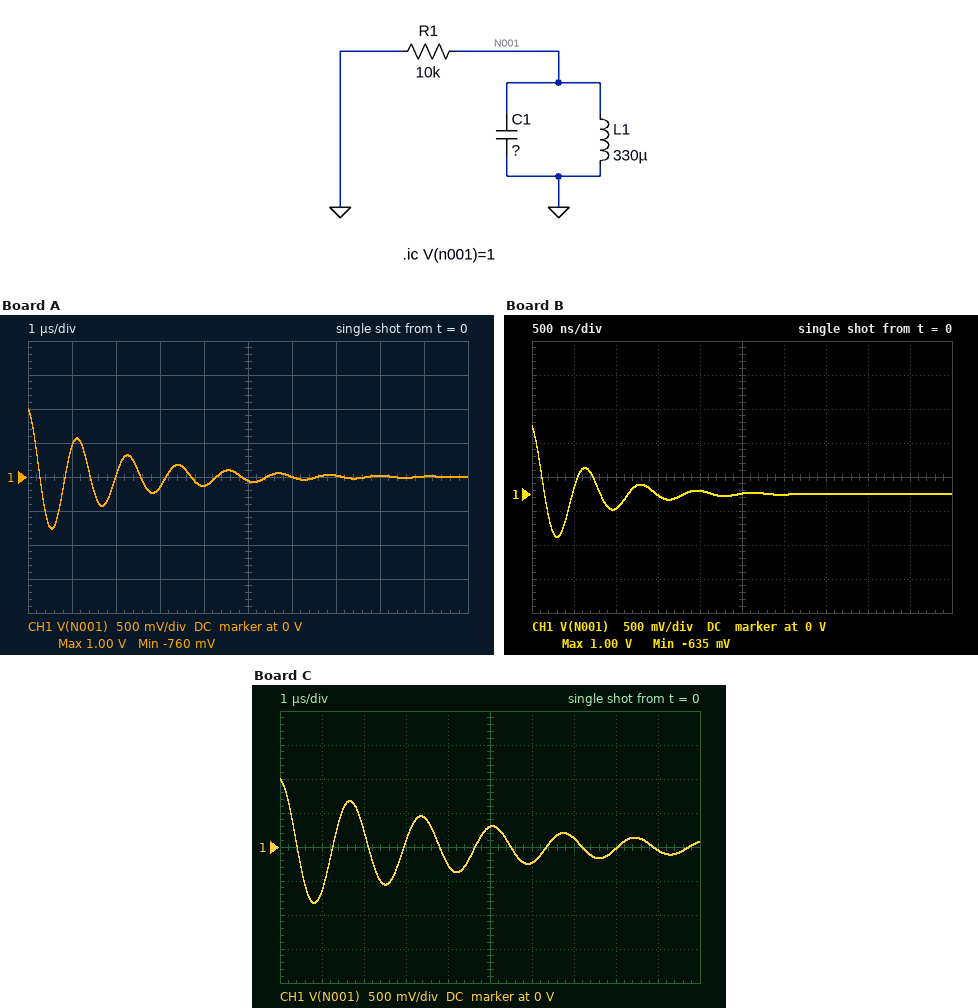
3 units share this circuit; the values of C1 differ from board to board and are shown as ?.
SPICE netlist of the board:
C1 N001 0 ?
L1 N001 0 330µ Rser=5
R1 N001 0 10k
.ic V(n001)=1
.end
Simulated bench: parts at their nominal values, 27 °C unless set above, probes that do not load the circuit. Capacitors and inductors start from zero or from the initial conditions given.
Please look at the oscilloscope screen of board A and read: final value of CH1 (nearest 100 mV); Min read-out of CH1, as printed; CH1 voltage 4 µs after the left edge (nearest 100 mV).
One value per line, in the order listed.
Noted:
0 V
-760 mV
-100 mV
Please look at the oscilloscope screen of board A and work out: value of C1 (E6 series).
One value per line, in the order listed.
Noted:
100 pF
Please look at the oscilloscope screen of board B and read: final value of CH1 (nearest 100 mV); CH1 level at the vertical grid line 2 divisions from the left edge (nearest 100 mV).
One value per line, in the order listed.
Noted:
0 V
-200 mV
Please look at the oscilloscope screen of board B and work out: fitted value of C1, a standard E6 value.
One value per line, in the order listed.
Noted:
33 pF
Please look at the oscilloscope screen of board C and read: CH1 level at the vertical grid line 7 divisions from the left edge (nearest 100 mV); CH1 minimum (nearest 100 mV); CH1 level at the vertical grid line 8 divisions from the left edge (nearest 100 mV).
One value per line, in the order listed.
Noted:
100 mV
-800 mV
0 V
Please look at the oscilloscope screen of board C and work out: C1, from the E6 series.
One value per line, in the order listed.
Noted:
220 pF
